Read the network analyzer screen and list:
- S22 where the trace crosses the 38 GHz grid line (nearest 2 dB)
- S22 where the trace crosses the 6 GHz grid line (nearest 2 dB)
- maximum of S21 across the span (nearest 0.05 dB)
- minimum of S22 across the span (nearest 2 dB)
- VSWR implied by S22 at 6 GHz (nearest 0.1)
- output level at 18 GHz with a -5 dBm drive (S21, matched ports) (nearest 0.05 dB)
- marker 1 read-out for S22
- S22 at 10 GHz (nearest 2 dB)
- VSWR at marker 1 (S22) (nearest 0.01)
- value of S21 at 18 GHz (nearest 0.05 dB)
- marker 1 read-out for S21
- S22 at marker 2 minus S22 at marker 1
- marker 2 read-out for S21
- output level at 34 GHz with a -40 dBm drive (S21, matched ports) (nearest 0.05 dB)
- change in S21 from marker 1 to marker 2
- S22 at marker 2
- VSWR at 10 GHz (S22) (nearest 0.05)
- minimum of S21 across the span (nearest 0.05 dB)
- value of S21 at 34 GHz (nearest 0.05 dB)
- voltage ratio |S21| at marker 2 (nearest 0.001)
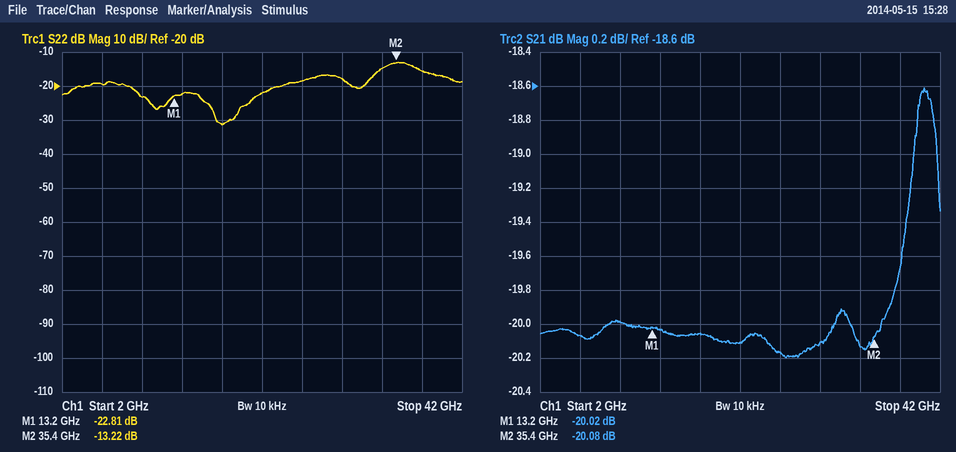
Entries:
-16 dB
-20 dB
-18.60 dB
-32 dB
1.2
-25.05 dBm
-22.81 dB
-24 dB
1.16
-20.05 dB
-20.02 dB
9.59 dB
-20.08 dB
-60.15 dBm
-0.06 dB
-13.22 dB
1.15
-20.20 dB
-20.15 dB
0.099
